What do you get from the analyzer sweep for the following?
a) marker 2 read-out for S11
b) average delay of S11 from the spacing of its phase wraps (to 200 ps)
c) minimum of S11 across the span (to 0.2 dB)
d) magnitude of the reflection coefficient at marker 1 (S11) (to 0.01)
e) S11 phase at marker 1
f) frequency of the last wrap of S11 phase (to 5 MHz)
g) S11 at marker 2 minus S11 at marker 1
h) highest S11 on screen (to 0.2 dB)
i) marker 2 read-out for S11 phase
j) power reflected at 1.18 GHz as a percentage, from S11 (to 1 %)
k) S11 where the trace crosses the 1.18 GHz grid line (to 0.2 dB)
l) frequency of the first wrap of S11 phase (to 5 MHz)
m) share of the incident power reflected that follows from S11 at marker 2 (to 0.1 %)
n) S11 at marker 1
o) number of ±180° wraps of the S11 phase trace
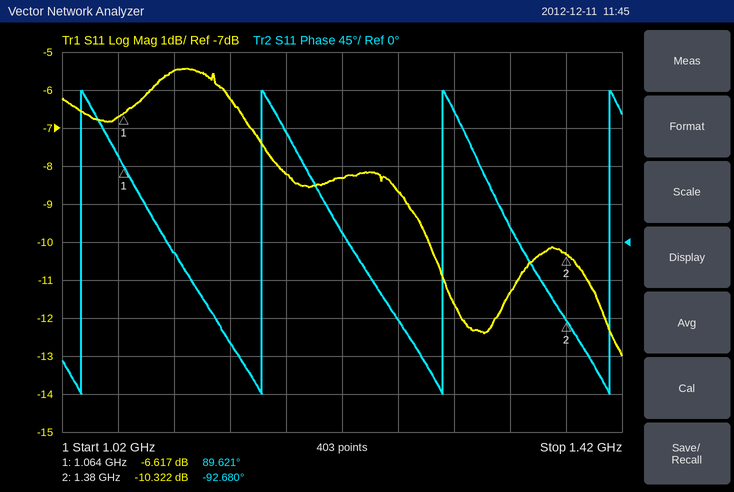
-10.322 dB
8.0 ns
-13.0 dB
0.47
89.621°
1.410 GHz
-3.705 dB
-5.4 dB
-92.680°
15 %
-8.2 dB
1.035 GHz
9.3 %
-6.617 dB
4
